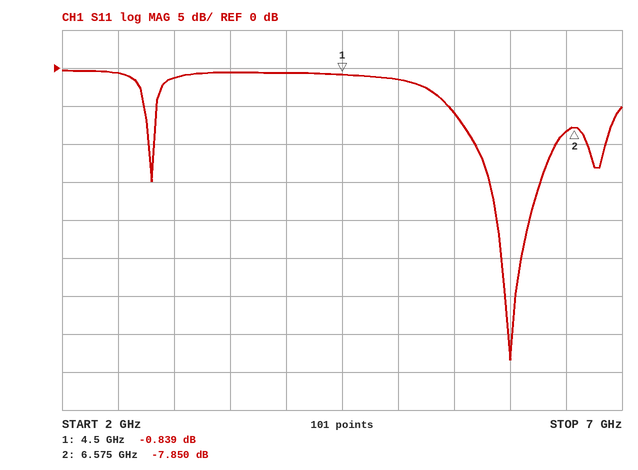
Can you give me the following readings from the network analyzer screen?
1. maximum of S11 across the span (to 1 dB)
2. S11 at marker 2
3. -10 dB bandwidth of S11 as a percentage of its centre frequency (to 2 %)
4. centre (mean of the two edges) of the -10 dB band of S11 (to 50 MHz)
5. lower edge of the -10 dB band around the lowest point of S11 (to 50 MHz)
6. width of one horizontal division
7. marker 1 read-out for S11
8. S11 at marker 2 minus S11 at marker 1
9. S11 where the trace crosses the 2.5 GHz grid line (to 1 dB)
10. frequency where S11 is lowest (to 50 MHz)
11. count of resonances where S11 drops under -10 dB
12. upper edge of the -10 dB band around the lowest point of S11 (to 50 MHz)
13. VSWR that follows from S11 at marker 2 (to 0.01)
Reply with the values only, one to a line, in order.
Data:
0 dB
-7.850 dB
12 %
6.05 GHz
5.70 GHz
500 MHz
-0.839 dB
-7.011 dB
-1 dB
6.00 GHz
3
6.40 GHz
2.36
